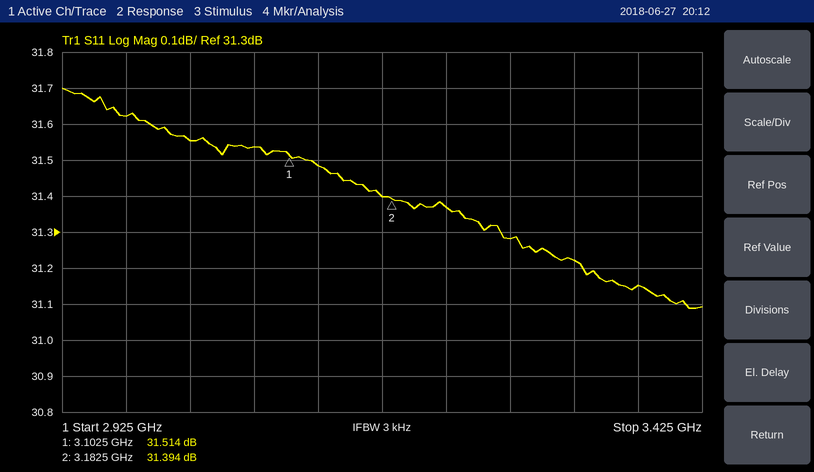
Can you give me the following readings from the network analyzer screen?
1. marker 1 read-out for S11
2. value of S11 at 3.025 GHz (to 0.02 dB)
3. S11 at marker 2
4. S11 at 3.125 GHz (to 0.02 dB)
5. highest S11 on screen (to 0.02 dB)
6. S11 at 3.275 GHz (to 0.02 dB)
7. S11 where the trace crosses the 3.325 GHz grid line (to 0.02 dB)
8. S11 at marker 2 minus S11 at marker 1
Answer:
31.514 dB
31.56 dB
31.394 dB
31.48 dB
31.70 dB
31.28 dB
31.22 dB
-0.120 dB
